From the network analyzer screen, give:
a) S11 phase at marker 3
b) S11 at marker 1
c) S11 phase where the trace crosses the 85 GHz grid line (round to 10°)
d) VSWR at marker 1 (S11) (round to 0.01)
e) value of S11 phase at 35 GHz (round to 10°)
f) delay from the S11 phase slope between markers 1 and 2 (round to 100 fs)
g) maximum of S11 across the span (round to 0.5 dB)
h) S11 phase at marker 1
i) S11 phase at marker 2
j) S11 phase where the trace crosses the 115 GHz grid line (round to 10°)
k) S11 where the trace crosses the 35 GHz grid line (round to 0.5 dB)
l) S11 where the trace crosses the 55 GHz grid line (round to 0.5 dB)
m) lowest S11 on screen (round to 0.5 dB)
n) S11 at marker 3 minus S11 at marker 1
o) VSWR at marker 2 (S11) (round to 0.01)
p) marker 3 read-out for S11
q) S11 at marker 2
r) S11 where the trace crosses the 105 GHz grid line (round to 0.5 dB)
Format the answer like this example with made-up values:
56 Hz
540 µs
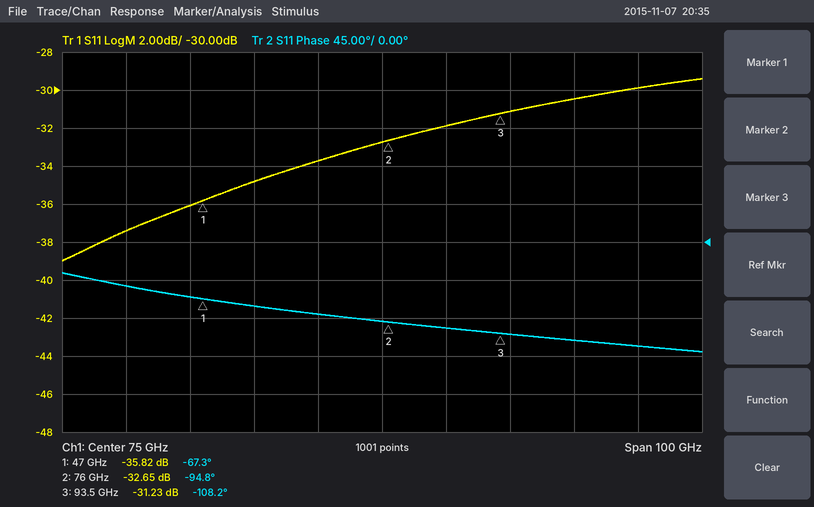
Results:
-108.2°
-35.82 dB
-100°
1.03
-50°
2.6 ps
-29.5 dB
-67.3°
-94.8°
-120°
-37.5 dB
-35.0 dB
-39.0 dB
4.59 dB
1.05
-31.23 dB
-32.65 dB
-30.5 dB
